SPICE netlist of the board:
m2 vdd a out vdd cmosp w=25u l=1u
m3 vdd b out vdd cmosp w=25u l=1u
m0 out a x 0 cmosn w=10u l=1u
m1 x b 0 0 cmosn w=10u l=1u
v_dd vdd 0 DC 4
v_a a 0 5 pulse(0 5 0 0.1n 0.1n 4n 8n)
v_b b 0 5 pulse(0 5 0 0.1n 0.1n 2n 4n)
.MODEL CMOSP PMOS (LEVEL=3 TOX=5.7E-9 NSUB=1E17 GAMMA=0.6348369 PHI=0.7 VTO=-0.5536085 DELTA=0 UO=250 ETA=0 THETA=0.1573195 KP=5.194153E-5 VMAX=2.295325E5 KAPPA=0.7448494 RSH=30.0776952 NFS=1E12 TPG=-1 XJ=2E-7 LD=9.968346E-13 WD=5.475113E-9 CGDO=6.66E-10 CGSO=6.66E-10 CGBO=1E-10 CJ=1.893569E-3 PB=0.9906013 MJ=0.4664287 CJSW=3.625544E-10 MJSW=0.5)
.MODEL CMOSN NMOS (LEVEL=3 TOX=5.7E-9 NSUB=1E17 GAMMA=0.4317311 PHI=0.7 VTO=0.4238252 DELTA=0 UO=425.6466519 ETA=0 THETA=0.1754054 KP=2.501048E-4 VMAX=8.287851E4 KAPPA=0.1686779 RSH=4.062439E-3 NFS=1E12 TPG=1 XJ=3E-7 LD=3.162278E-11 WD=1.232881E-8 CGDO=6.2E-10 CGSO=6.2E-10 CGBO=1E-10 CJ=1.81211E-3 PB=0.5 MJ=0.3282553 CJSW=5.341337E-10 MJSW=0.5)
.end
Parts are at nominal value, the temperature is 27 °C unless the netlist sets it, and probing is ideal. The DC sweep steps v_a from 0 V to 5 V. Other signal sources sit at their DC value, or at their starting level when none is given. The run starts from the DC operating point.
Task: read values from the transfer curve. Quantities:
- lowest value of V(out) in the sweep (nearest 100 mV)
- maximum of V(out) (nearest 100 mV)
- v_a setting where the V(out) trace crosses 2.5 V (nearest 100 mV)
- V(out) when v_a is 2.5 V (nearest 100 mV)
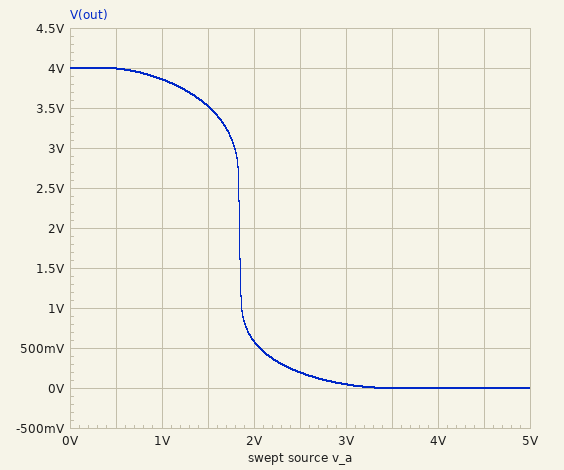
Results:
0 V
4.0 V
1.8 V
200 mV
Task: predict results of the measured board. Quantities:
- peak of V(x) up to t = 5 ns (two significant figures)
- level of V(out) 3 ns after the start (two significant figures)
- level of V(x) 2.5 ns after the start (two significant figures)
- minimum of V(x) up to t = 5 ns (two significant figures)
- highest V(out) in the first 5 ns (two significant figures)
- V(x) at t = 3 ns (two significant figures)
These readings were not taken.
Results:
4.1 V
4.0 V
3.7 V
-630 mV
4.7 V
4.0 V
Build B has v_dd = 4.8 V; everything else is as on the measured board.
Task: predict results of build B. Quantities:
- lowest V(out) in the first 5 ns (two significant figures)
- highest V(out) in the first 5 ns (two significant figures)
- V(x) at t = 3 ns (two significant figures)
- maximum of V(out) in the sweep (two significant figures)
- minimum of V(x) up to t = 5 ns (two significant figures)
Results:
-430 mV
5.5 V
4.1 V
4.8 V
-500 mV
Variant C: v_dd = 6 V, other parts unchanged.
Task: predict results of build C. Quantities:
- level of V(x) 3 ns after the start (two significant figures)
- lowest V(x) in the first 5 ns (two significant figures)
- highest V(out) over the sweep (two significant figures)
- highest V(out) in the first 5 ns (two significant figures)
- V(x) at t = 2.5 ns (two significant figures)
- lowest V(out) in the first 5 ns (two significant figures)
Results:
4.1 V
-320 mV
6.0 V
6.7 V
4.0 V
-170 mV
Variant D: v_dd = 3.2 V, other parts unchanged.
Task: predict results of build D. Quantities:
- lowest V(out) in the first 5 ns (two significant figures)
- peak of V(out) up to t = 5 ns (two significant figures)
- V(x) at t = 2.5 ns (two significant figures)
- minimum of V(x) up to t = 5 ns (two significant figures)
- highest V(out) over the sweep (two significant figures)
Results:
-670 mV
3.9 V
2.9 V
-650 mV
3.2 V
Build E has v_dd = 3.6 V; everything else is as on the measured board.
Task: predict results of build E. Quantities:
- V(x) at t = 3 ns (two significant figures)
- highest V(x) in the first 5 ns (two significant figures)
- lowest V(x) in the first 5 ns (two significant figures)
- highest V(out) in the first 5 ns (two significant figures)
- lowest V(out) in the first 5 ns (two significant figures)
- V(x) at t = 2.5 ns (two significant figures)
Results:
3.6 V
3.8 V
-640 mV
4.3 V
-660 mV
3.3 V
